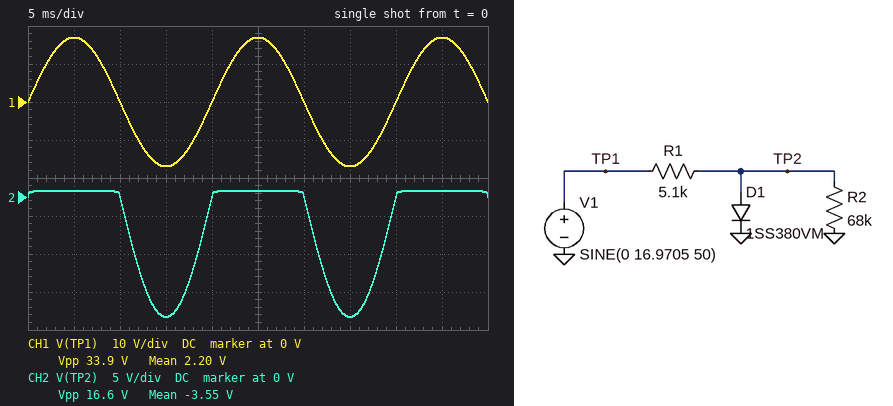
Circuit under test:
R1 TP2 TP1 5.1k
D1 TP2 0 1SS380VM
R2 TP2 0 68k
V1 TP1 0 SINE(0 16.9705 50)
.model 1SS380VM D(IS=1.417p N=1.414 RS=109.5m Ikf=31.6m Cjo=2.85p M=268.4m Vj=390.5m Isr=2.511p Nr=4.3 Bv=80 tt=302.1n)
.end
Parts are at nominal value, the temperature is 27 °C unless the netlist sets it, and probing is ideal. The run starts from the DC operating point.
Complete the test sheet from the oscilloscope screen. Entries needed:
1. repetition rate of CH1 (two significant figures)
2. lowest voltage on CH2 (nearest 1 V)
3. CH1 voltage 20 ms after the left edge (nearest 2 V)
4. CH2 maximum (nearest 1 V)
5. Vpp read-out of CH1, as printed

50 Hz
-16 V
0 V
1 V
33.9 V
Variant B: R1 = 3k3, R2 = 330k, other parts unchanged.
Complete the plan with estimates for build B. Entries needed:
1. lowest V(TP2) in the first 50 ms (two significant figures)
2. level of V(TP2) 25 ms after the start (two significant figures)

-17 V
820 mV
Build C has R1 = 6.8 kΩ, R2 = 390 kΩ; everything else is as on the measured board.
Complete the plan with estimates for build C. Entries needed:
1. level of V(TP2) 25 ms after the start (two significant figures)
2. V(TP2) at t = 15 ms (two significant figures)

790 mV
-17 V
